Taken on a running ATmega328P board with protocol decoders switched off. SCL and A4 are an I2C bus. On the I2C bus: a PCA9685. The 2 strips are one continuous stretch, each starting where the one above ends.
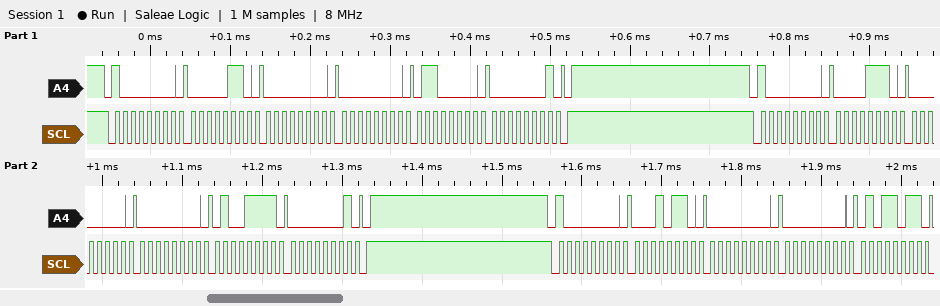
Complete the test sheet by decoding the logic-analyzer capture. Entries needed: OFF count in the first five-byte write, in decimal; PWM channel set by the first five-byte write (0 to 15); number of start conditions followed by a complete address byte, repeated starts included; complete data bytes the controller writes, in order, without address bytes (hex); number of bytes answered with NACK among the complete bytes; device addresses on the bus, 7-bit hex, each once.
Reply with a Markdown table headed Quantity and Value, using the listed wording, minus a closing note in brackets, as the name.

| Quantity | Value |
|---|---|
| OFF count in the first five-byte write, in decimal | 352 |
| PWM channel set by the first five-byte write | 0 |
| number of start conditions followed by a complete address byte, repeated starts included | 3 |
| complete data bytes the controller writes, in order, without address bytes | 06 00 00 60 01 0E 00 00 4F 01 16 00 00 5B |
| number of bytes answered with NACK among the complete bytes | 0 |
| device addresses on the bus, 7-bit hex, each once | 0x40 |
